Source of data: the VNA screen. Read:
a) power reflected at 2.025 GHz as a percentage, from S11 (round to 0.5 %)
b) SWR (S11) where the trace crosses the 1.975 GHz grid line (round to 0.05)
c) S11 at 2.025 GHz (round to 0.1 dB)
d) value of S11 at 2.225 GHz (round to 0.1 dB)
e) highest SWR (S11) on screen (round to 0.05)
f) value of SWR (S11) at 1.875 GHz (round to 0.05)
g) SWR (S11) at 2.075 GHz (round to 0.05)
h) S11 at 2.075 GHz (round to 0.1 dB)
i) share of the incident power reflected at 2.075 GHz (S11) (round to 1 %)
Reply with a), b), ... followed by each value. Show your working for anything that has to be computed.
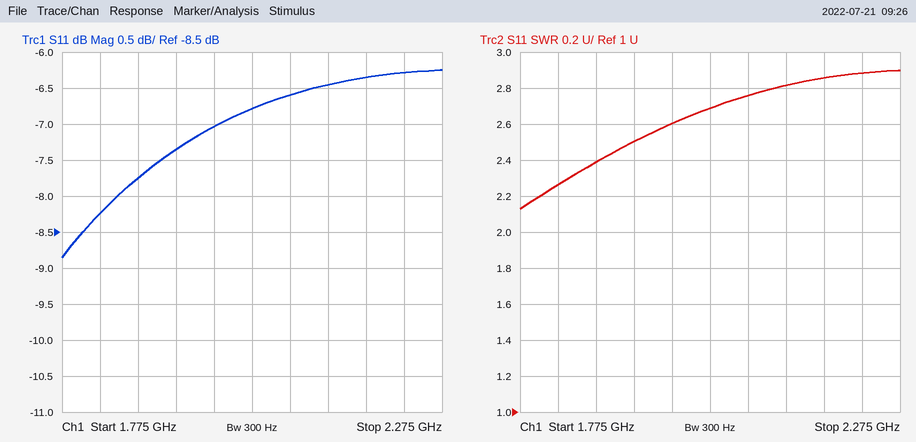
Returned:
a) 10^(-6.8/10) ≈ 20.9 %, so 21.0 % to the nearest 0.5 %
b) 2.60
c) -6.8 dB
d) -6.3 dB
e) 2.90
f) 2.40
g) 2.75
h) -6.6 dB
i) 10^(-6.6/10) ≈ 22 %
